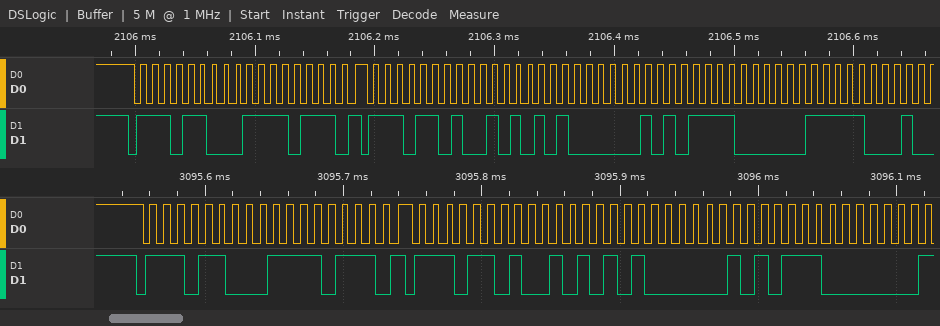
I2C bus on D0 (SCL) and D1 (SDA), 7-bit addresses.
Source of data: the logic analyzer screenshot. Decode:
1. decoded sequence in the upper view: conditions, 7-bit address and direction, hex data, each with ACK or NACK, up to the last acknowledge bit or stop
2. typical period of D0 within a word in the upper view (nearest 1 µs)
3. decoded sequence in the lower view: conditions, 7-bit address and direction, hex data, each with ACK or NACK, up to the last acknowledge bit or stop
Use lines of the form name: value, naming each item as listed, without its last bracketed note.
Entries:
decoded sequence in the upper view: conditions, 7-bit address and direction, hex data, each with ACK or NACK, up to the last acknowledge bit or stop: start, address 76 write ACK, F7 ACK, repeated start, address 76 read ACK, 55 ACK, 05 ACK, F0 ACK, 7C ACK
typical period of D0 within a word in the upper view: 10 µs
decoded sequence in the lower view: conditions, 7-bit address and direction, hex data, each with ACK or NACK, up to the last acknowledge bit or stop: start, address 76 write ACK, F7 ACK, repeated start, address 76 read ACK, 55 ACK, 05 ACK, E0 ACK
